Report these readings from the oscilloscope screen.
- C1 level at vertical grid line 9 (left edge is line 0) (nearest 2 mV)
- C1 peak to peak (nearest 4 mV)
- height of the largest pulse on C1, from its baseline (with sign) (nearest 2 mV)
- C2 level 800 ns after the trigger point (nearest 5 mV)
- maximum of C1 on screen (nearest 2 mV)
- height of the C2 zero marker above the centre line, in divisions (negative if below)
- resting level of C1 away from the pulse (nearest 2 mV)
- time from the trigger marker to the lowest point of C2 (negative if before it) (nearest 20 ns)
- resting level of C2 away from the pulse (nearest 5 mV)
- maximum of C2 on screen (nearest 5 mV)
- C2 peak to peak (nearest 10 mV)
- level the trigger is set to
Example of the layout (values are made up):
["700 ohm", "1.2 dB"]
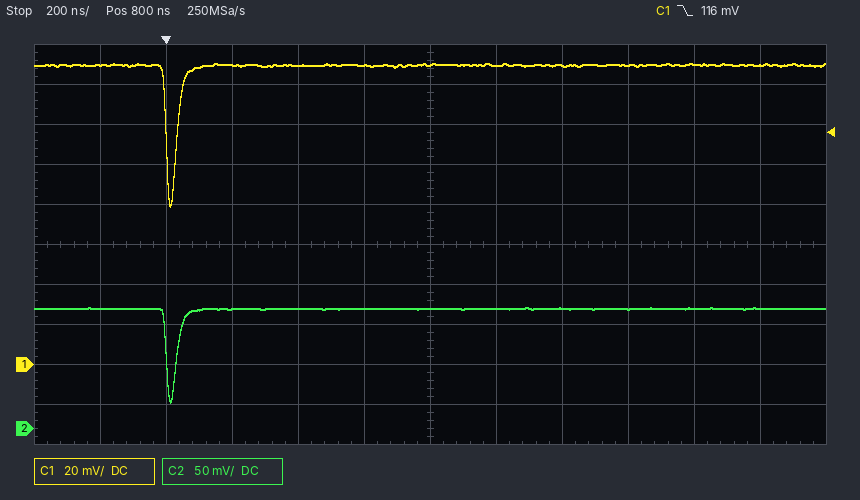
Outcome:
["150 mV", "72 mV", "-70 mV", "150 mV", "150 mV", "-4.6 div", "150 mV", "+20 ns", "150 mV", "150 mV", "120 mV", "116 mV"]
